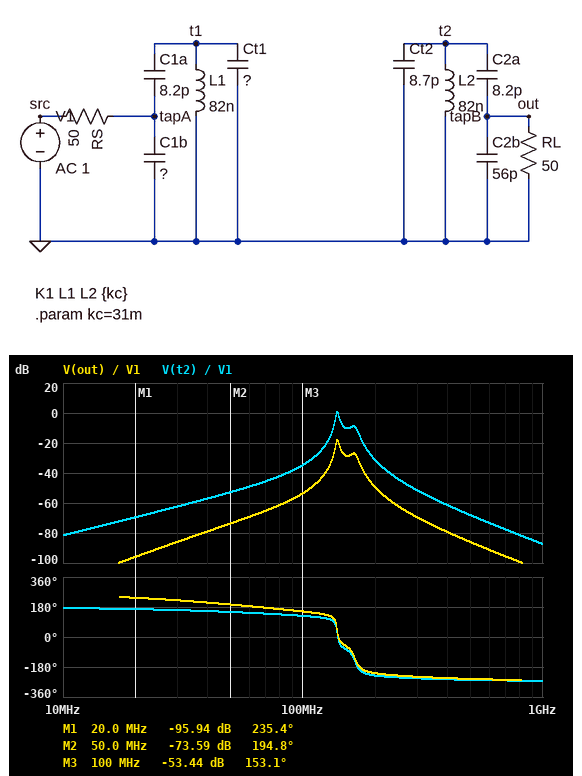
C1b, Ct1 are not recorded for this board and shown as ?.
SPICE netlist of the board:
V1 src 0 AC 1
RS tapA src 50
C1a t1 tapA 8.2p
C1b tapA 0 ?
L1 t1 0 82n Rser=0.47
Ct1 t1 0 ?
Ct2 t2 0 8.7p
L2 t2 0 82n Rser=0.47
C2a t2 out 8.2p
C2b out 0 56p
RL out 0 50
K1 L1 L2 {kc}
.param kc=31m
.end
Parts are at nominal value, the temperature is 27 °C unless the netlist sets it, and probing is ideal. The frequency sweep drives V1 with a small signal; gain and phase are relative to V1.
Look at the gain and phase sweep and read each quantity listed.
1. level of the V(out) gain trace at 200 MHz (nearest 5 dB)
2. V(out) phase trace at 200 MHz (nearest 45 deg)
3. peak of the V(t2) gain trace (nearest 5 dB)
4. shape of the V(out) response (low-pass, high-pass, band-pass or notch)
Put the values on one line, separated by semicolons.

-50 dB; -225 deg; 0 dB; band-pass
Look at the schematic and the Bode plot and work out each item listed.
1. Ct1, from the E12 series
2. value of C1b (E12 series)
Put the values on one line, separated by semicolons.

4.7 pF; 27 pF
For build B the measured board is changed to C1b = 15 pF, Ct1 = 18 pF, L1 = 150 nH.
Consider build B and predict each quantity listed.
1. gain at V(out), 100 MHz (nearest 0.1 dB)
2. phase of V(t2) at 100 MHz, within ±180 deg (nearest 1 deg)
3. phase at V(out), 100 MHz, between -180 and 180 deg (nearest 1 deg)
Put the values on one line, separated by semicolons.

-47.4 dB; -28 deg; -2 deg
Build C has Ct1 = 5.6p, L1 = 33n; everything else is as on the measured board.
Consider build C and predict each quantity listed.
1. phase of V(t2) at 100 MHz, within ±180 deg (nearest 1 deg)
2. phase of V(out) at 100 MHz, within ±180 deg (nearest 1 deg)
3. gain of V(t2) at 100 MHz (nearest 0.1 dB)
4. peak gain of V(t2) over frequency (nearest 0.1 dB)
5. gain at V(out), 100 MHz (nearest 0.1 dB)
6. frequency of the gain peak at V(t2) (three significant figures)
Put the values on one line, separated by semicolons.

129 deg; 155 deg; -41.2 dB; -10.7 dB; -60.0 dB; 139 MHz
